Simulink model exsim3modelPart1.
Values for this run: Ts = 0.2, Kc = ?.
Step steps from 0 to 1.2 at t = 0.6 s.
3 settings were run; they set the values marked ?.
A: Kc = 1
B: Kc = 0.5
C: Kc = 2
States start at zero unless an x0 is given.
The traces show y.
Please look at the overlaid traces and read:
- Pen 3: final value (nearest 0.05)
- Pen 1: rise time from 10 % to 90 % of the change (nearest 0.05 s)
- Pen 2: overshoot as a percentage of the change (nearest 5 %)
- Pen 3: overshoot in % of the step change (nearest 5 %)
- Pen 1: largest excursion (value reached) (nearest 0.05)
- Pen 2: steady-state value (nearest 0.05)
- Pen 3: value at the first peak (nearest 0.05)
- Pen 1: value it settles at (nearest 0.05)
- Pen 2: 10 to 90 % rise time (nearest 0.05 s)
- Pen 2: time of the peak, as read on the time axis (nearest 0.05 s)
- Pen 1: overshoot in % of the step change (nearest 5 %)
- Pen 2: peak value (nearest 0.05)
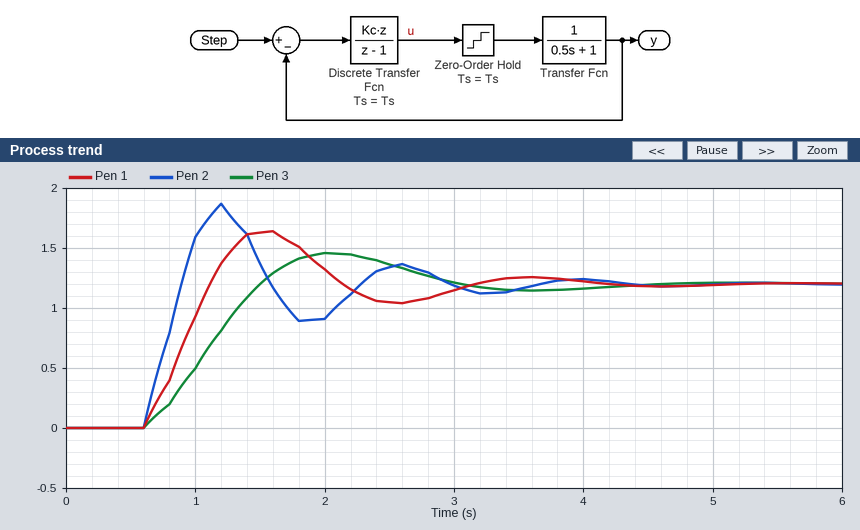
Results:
1.20
0.40 s
55 %
20 %
1.65
1.20
1.45
1.20
0.25 s
1.20 s
35 %
1.85
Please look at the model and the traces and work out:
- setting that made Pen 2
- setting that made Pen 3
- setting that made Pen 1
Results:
C
B
A
